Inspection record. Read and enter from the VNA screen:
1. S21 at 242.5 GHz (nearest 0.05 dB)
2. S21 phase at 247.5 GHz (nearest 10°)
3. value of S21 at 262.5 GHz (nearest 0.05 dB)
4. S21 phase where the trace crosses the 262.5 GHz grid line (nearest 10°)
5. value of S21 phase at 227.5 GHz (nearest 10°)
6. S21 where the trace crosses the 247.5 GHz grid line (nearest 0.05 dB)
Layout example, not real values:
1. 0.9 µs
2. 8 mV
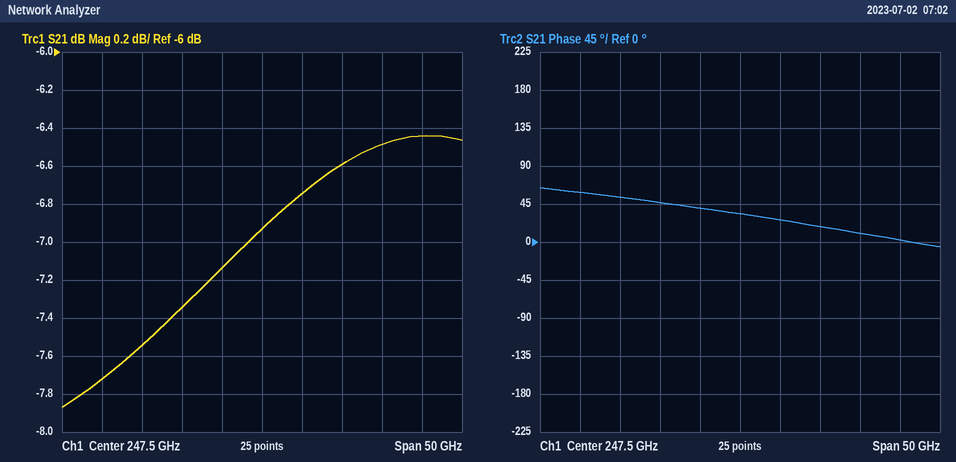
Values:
1. -7.15 dB
2. 30°
3. -6.50 dB
4. 10°
5. 60°
6. -6.95 dB
